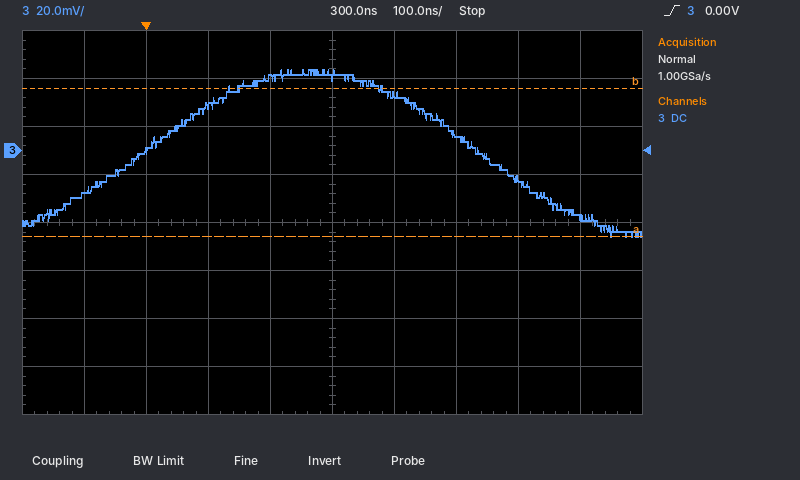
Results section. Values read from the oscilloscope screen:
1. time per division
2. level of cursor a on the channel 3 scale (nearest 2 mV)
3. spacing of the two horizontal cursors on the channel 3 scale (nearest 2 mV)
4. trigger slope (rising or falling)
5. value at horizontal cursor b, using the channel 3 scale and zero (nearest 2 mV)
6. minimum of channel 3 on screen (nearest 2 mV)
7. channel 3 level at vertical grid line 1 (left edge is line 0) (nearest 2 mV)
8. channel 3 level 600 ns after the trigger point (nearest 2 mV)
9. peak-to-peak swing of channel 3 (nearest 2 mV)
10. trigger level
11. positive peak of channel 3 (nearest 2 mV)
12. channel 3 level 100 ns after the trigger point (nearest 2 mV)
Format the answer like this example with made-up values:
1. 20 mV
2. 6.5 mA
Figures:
1. 100 ns
2. -36 mV
3. 62 mV
4. rising
5. 26 mV
6. -36 mV
7. -18 mV
8. -12 mV
9. 70 mV
10. 0.00 V
11. 34 mV
12. 18 mV
